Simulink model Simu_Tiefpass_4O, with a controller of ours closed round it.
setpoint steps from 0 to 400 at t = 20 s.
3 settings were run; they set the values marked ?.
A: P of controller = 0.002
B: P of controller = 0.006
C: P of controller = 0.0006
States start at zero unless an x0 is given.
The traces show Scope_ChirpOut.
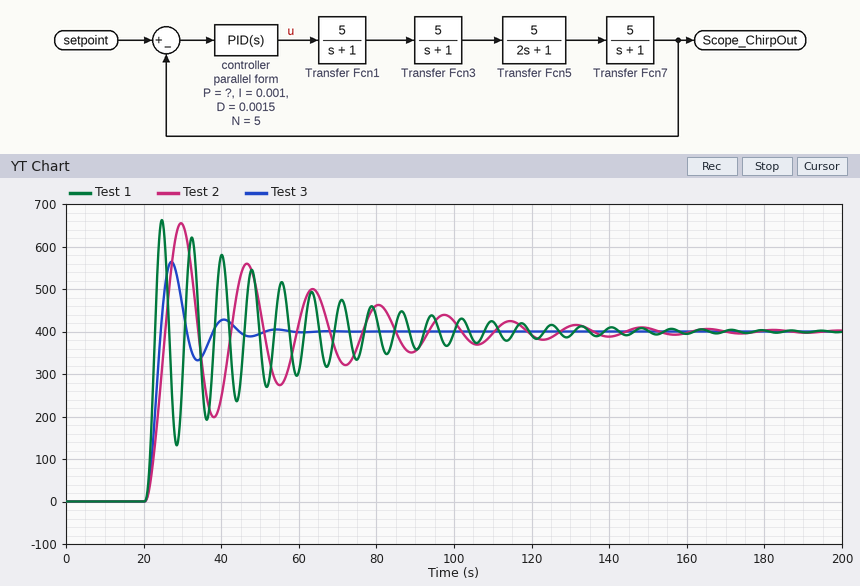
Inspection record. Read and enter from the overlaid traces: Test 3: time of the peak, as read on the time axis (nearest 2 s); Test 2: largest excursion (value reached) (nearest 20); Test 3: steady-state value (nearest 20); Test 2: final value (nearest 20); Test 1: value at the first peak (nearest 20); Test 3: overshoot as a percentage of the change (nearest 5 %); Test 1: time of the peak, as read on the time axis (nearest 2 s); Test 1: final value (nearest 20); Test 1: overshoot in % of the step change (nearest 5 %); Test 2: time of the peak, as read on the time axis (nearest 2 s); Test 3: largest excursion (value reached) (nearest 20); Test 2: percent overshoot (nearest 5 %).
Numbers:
28 s
660
400
400
660
40 %
24 s
400
65 %
30 s
560
65 %
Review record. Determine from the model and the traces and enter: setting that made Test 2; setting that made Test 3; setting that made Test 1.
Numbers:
C
A
B
